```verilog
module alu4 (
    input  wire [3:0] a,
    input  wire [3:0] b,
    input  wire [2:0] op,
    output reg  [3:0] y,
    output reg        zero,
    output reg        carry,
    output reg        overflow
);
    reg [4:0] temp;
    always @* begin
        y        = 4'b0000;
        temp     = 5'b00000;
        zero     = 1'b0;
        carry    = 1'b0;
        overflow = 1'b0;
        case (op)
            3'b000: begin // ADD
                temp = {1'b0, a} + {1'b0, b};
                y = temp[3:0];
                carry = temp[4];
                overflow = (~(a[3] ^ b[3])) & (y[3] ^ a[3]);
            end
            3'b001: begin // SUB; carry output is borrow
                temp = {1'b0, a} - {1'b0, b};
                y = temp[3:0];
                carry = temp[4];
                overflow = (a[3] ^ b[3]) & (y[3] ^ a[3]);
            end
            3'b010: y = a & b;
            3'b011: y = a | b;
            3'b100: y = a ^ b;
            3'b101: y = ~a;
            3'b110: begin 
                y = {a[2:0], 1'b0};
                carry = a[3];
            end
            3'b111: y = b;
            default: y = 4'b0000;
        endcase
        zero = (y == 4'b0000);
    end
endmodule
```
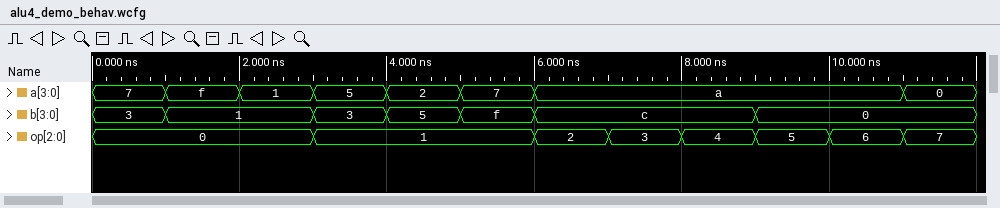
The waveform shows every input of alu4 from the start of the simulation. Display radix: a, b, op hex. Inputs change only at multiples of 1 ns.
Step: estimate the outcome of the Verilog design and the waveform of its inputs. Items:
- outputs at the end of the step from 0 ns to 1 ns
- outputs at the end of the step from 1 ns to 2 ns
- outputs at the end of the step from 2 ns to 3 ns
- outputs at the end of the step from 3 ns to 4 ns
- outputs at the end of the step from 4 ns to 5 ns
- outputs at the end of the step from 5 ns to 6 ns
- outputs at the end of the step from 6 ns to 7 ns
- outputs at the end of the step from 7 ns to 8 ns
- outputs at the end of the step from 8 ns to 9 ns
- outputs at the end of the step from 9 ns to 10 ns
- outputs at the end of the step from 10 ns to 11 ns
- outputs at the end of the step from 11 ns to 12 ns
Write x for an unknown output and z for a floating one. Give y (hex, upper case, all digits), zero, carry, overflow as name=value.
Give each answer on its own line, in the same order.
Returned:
y=A, zero=0, carry=0, overflow=1
y=0, zero=1, carry=1, overflow=0
y=2, zero=0, carry=0, overflow=0
y=2, zero=0, carry=0, overflow=0
y=D, zero=0, carry=1, overflow=0
y=8, zero=0, carry=1, overflow=1
y=8, zero=0, carry=0, overflow=0
y=E, zero=0, carry=0, overflow=0
y=6, zero=0, carry=0, overflow=0
y=5, zero=0, carry=0, overflow=0
y=4, zero=0, carry=1, overflow=0
y=0, zero=1, carry=0, overflow=0
